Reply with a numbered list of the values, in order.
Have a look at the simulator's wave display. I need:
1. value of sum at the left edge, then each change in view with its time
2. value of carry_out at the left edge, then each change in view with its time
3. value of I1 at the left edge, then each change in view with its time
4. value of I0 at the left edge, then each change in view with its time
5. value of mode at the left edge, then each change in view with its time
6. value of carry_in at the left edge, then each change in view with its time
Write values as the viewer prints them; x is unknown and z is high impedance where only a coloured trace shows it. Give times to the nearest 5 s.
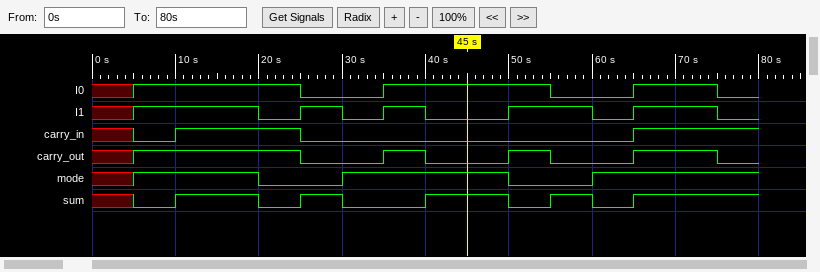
1. x, 0 at 5 s, 1 at 10 s, 0 at 20 s, 1 at 25 s, 0 at 30 s, 1 at 40 s, 0 at 50 s, 1 at 55 s, 0 at 60 s, 1 at 65 s
2. x, 1 at 5 s, 0 at 25 s, 1 at 35 s, 0 at 40 s, 1 at 50 s, 0 at 55 s, 1 at 65 s, 0 at 75 s
3. x, 1 at 5 s, 0 at 20 s, 1 at 25 s, 0 at 30 s, 1 at 35 s, 0 at 40 s, 1 at 50 s, 0 at 60 s, 1 at 65 s, 0 at 75 s
4. x, 1 at 5 s, 0 at 25 s, 1 at 35 s, 0 at 55 s, 1 at 65 s, 0 at 75 s
5. x, 1 at 5 s, 0 at 20 s, 1 at 30 s, 0 at 50 s, 1 at 60 s
6. x, 0 at 5 s, 1 at 10 s, 0 at 25 s, 1 at 65 s
